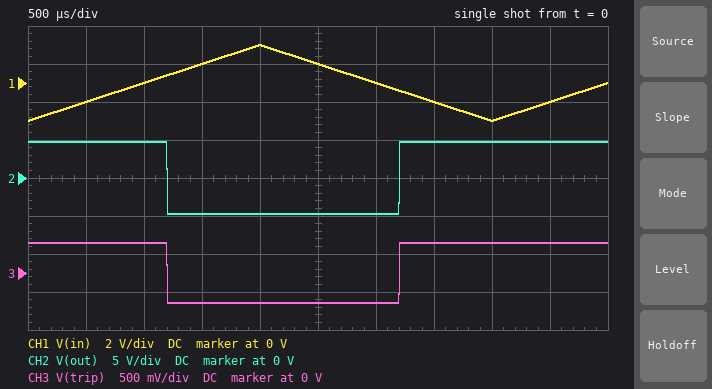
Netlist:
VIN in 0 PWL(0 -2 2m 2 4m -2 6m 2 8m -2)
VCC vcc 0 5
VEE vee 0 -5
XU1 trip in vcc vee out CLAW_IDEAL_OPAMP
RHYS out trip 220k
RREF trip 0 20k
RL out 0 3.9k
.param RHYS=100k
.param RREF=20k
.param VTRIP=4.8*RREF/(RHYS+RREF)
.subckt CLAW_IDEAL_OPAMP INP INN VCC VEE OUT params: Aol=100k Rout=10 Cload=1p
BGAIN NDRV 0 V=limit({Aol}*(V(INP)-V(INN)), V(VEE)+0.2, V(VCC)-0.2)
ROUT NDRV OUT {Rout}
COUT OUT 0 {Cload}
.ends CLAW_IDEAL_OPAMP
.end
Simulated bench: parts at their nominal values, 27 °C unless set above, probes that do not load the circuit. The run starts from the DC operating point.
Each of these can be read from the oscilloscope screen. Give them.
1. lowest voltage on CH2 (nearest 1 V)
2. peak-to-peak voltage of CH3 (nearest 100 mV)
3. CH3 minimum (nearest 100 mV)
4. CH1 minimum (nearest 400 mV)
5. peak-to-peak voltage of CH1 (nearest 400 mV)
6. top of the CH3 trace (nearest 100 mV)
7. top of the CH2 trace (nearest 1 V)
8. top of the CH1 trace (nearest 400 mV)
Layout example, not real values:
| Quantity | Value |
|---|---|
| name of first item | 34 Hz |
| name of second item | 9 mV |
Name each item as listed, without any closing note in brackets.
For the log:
| Quantity | Value |
|---|---|
| lowest voltage on CH2 | -5 V |
| peak-to-peak voltage of CH3 | 800 mV |
| CH3 minimum | -400 mV |
| CH1 minimum | -2.0 V |
| peak-to-peak voltage of CH1 | 4.0 V |
| top of the CH3 trace | 400 mV |
| top of the CH2 trace | 5 V |
| top of the CH1 trace | 2.0 V |
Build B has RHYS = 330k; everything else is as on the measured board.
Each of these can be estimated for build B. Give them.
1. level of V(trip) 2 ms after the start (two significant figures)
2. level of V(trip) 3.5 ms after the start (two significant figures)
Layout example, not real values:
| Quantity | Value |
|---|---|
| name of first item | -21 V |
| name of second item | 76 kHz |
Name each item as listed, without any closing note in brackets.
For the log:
| Quantity | Value |
|---|---|
| level of V(trip) 2 ms after the start | -270 mV |
| level of V(trip) 3.5 ms after the start | 270 mV |
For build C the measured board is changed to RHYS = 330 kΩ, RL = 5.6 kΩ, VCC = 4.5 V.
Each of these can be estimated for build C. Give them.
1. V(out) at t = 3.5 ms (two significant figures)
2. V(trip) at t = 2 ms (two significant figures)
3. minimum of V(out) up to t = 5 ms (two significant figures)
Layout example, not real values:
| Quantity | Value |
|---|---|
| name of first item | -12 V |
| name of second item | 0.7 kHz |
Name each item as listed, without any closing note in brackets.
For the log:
| Quantity | Value |
|---|---|
| V(out) at t = 3.5 ms | 4.3 V |
| V(trip) at t = 2 ms | -270 mV |
| minimum of V(out) up to t = 5 ms | -4.8 V |
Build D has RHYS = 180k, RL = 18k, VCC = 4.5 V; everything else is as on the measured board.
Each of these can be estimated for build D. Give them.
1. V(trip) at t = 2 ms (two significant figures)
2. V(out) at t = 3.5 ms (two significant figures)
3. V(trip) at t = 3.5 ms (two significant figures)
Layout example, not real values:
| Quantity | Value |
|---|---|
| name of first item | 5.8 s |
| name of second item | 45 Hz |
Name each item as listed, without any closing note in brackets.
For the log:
| Quantity | Value |
|---|---|
| V(trip) at t = 2 ms | -480 mV |
| V(out) at t = 3.5 ms | 4.3 V |
| V(trip) at t = 3.5 ms | 430 mV |
